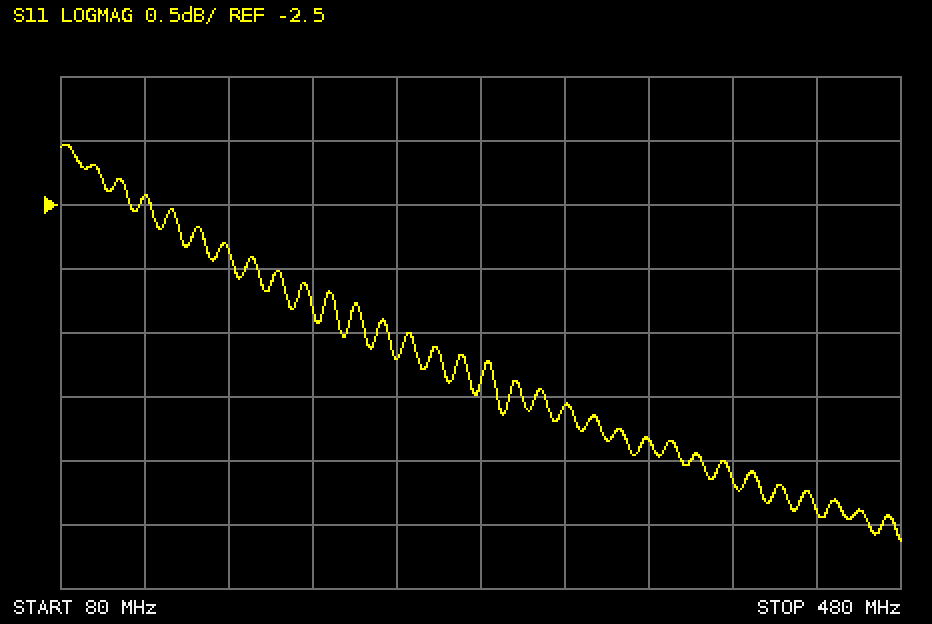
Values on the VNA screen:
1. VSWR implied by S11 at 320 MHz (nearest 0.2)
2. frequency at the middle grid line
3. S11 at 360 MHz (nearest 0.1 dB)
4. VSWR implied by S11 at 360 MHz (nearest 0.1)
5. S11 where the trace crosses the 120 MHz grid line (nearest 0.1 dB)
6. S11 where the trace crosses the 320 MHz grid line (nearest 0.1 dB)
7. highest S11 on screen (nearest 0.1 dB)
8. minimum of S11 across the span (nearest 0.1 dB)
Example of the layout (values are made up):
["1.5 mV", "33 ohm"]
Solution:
["4.4", "280 MHz", "-4.3 dB", "4.1", "-2.4 dB", "-4.1 dB", "-2.0 dB", "-5.1 dB"]
